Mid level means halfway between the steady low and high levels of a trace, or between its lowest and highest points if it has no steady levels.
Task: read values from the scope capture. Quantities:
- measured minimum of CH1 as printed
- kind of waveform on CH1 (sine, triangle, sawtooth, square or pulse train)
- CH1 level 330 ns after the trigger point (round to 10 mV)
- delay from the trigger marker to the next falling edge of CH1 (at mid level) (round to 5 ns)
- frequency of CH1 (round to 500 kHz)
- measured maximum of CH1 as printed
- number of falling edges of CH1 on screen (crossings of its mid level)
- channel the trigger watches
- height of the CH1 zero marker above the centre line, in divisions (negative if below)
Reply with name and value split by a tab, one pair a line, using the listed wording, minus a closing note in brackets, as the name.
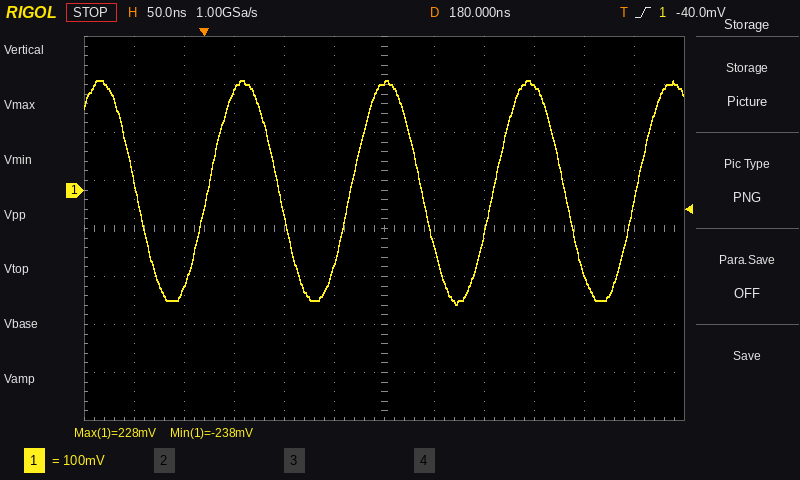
measured minimum of CH1 as printed	-238 mV
kind of waveform on CH1	sine
CH1 level 330 ns after the trigger point	220 mV
delay from the trigger marker to the next falling edge of CH1 (at mid level)	75 ns
frequency of CH1	7.0 MHz
measured maximum of CH1 as printed	228 mV
number of falling edges of CH1 on screen	4
channel the trigger watches	CH1
height of the CH1 zero marker above the centre line, in divisions	+0.8 div
